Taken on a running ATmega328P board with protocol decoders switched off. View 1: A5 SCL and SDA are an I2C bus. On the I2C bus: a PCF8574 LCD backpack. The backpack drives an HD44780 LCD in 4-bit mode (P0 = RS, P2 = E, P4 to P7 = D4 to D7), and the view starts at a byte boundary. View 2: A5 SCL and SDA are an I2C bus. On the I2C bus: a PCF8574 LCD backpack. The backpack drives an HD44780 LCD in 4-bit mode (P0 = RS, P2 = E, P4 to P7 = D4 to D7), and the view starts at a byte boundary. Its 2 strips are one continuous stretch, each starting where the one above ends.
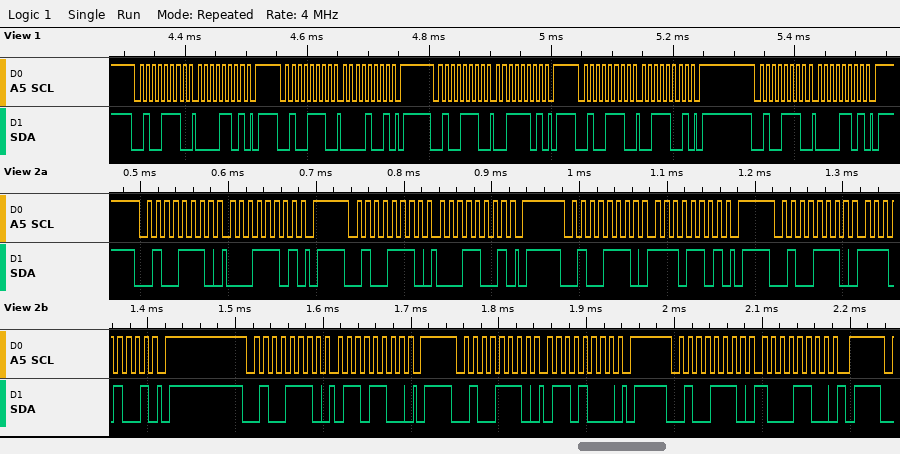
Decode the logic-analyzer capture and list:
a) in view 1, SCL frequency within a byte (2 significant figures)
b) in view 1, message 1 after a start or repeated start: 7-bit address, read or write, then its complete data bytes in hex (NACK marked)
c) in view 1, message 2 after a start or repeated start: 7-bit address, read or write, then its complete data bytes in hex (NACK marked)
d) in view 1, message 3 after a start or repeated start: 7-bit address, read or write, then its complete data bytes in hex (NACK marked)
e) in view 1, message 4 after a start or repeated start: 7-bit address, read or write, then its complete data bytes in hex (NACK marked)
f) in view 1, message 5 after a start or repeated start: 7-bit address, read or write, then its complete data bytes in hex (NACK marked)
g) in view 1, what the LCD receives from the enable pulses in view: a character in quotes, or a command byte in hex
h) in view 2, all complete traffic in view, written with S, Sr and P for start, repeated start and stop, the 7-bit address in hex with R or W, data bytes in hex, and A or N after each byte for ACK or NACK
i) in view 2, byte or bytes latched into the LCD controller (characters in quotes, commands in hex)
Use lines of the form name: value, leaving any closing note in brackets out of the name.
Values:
in view 1, SCL frequency within a byte: 100 kHz
in view 1, message 1 after a start or repeated start: 7-bit address, read or write, then its complete data bytes in hex: 0x27 write: 0D
in view 1, message 2 after a start or repeated start: 7-bit address, read or write, then its complete data bytes in hex: 0x27 write: 09
in view 1, message 3 after a start or repeated start: 7-bit address, read or write, then its complete data bytes in hex: 0x27 write: 3D
in view 1, message 4 after a start or repeated start: 7-bit address, read or write, then its complete data bytes in hex: 0x27 write: 39
in view 1, message 5 after a start or repeated start: 7-bit address, read or write, then its complete data bytes in hex: 0x27 write: 0D
in view 1, what the LCD receives from the enable pulses in view: a character in quotes, or a command byte in hex: data 0x03
in view 2, all complete traffic in view, written with S, Sr and P for start, repeated start and stop, the 7-bit address in hex with R or W, data bytes in hex, and A or N after each byte for ACK or NACK: S 27W A 1D A P S 27W A 19 A P S 27W A ED A P S 27W A E9 A P S 27W A 6C A P S 27W A 68 A P S 27W A 8C A P
in view 2, byte or bytes latched into the LCD controller: data 0x1E
